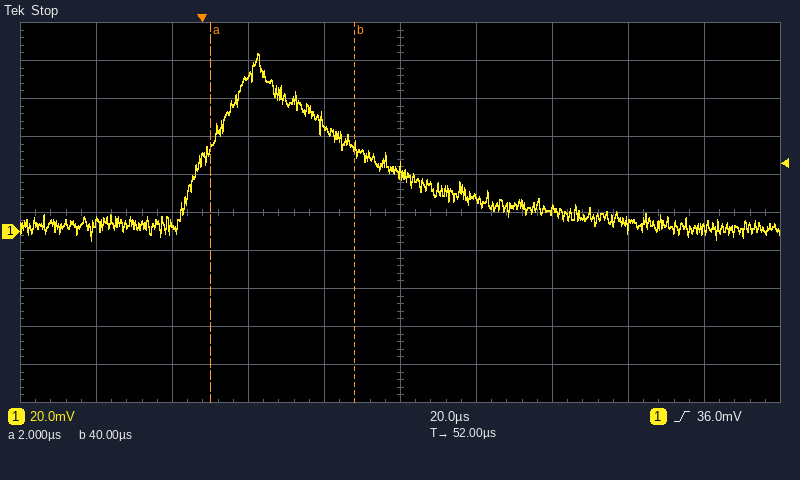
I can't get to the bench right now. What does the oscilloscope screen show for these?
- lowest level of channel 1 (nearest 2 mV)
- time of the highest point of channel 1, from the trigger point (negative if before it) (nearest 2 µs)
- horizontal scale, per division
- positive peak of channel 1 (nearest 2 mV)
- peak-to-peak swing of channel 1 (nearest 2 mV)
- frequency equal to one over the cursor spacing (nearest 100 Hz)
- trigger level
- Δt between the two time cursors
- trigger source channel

-4 mV
+14 µs
20 µs
94 mV
98 mV
26.3 kHz
36.0 mV
38 µs
channel 1
